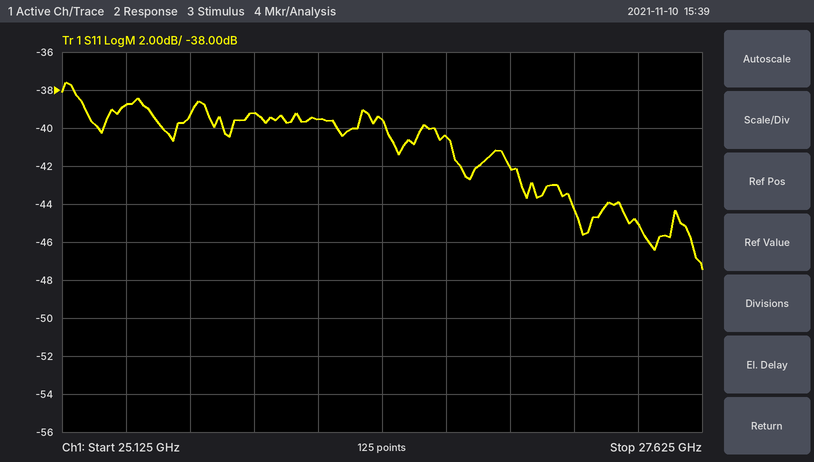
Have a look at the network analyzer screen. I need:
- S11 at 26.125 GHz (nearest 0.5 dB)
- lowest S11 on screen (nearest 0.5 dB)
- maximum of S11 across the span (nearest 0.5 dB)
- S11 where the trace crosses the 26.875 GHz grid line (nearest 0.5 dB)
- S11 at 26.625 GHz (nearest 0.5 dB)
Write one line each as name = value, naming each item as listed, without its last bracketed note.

S11 at 26.125 GHz = -39.5 dB
lowest S11 on screen = -47.5 dB
maximum of S11 across the span = -37.5 dB
S11 where the trace crosses the 26.875 GHz grid line = -42.0 dB
S11 at 26.625 GHz = -40.5 dB
